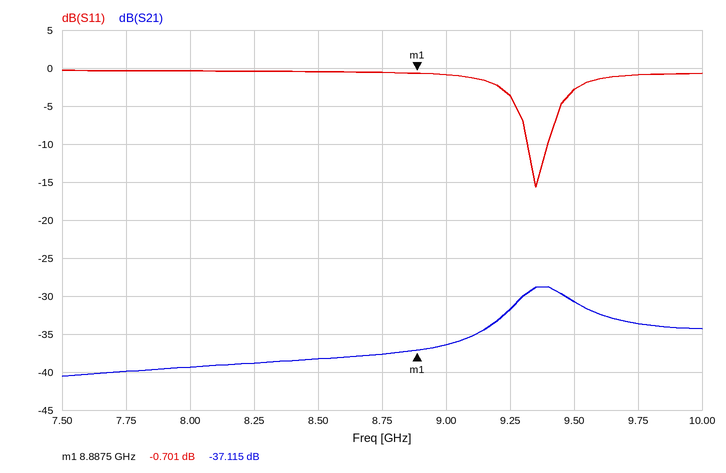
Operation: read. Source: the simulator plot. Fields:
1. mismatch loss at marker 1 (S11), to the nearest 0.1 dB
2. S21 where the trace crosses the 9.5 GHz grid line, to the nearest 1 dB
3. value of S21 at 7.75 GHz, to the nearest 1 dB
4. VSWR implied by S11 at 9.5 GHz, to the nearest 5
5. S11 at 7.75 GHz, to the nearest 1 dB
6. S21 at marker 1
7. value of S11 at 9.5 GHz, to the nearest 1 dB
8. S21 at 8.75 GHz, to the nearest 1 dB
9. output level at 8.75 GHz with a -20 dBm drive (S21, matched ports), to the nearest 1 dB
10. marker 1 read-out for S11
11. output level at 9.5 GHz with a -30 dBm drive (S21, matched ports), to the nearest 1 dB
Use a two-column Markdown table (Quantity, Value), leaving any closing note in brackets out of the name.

| Quantity | Value |
|---|---|
| mismatch loss at marker 1 (S11), to the nearest 0.1 dB | 8.3 dB |
| S21 where the trace crosses the 9.5 GHz grid line, to the nearest 1 dB | -31 dB |
| value of S21 at 7.75 GHz, to the nearest 1 dB | -40 dB |
| VSWR implied by S11 at 9.5 GHz, to the nearest 5 | 5 |
| S11 at 7.75 GHz, to the nearest 1 dB | 0 dB |
| S21 at marker 1 | -37.115 dB |
| value of S11 at 9.5 GHz, to the nearest 1 dB | -3 dB |
| S21 at 8.75 GHz, to the nearest 1 dB | -38 dB |
| output level at 8.75 GHz with a -20 dBm drive (S21, matched ports), to the nearest 1 dB | -58 dBm |
| marker 1 read-out for S11 | -0.701 dB |
| output level at 9.5 GHz with a -30 dBm drive (S21, matched ports), to the nearest 1 dB | -61 dBm |
